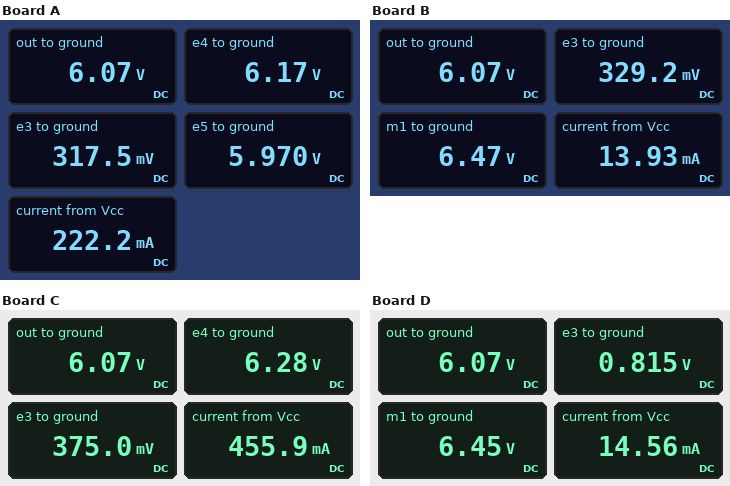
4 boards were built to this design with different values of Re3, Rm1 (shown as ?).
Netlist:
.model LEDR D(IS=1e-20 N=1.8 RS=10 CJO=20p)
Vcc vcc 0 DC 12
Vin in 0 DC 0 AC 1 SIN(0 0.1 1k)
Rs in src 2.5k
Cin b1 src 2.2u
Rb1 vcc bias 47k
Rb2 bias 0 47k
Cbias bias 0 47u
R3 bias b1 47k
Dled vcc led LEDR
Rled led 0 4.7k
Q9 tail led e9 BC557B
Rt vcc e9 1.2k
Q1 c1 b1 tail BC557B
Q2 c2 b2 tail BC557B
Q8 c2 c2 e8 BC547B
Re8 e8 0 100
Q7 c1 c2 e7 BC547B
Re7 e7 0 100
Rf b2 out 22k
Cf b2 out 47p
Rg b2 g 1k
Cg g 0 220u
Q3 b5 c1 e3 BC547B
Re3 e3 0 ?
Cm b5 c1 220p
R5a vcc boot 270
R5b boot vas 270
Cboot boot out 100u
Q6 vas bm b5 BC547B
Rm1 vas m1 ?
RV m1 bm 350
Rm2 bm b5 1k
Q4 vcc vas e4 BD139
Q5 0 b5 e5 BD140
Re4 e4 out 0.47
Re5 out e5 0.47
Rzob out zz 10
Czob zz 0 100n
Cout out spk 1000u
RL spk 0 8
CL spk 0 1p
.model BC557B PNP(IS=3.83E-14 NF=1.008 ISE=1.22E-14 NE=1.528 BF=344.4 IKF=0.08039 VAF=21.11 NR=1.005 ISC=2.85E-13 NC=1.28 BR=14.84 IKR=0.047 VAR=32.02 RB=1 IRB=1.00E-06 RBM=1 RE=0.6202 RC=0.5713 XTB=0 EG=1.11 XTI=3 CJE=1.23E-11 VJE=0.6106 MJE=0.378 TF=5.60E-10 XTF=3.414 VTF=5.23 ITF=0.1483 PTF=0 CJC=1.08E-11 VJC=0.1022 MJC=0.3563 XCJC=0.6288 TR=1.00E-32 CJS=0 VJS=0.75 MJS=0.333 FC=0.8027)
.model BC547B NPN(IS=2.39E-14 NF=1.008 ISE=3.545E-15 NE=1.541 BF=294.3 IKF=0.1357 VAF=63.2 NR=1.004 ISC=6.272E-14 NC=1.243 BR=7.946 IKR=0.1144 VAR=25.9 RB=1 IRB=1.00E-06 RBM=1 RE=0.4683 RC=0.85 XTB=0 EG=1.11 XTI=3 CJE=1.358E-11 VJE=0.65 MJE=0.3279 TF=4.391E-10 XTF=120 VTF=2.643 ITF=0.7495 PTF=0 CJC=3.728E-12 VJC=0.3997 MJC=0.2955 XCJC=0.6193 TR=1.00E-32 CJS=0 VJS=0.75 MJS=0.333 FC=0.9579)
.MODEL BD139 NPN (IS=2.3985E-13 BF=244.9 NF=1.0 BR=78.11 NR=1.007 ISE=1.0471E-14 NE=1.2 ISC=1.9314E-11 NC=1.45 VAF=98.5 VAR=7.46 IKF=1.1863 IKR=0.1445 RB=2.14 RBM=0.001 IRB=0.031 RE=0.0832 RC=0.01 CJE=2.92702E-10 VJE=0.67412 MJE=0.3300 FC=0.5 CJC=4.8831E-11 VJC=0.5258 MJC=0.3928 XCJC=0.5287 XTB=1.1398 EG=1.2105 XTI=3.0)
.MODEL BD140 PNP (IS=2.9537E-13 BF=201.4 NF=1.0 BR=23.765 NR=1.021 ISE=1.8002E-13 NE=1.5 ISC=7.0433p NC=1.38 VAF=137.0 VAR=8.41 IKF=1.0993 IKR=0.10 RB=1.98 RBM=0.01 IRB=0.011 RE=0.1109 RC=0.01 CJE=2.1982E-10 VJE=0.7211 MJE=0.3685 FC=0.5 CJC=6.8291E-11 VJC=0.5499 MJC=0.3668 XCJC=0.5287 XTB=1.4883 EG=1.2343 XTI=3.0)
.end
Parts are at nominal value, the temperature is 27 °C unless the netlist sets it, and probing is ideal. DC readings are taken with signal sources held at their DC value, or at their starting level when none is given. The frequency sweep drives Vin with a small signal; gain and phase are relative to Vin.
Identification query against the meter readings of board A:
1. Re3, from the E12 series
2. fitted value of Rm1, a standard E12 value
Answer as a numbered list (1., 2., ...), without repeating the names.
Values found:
1. 33 Ω
2. 1 kΩ
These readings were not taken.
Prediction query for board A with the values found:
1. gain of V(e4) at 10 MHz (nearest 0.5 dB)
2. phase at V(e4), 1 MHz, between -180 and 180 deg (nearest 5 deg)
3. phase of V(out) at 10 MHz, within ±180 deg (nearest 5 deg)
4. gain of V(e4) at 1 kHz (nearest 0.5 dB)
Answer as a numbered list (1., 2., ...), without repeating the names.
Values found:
1. -7.5 dB
2. -80 deg
3. 155 deg
4. 27.0 dB
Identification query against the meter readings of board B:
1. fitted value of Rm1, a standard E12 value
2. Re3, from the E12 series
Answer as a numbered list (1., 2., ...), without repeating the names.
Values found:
1. 220 Ω
2. 33 Ω
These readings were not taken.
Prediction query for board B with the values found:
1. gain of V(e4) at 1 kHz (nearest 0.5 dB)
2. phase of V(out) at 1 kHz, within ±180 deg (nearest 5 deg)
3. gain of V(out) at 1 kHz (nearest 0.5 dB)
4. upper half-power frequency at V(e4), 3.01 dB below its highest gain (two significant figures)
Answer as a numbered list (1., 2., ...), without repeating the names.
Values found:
1. 26.5 dB
2. 0 deg
3. 26.5 dB
4. 82 kHz
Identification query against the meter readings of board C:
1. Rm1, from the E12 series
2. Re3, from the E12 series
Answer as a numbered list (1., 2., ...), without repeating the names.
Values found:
1. 1.5 kΩ
2. 39 Ω
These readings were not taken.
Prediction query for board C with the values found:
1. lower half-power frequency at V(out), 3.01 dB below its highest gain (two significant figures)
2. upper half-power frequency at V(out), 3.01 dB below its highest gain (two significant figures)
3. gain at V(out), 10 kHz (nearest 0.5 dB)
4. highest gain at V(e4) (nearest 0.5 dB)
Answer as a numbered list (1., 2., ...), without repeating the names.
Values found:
1. 1.8 Hz
2. 120 kHz
3. 26.5 dB
4. 27.0 dB
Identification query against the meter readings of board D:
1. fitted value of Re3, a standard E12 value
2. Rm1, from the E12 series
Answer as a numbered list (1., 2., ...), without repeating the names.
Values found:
1. 82 Ω
2. 270 Ω
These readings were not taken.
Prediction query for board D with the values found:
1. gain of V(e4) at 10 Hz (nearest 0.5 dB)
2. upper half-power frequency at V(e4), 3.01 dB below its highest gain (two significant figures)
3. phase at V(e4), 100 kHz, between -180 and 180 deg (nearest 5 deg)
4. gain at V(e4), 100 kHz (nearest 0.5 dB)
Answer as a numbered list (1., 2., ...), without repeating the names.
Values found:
1. 26.5 dB
2. 95 kHz
3. -55 deg
4. 23.5 dB
